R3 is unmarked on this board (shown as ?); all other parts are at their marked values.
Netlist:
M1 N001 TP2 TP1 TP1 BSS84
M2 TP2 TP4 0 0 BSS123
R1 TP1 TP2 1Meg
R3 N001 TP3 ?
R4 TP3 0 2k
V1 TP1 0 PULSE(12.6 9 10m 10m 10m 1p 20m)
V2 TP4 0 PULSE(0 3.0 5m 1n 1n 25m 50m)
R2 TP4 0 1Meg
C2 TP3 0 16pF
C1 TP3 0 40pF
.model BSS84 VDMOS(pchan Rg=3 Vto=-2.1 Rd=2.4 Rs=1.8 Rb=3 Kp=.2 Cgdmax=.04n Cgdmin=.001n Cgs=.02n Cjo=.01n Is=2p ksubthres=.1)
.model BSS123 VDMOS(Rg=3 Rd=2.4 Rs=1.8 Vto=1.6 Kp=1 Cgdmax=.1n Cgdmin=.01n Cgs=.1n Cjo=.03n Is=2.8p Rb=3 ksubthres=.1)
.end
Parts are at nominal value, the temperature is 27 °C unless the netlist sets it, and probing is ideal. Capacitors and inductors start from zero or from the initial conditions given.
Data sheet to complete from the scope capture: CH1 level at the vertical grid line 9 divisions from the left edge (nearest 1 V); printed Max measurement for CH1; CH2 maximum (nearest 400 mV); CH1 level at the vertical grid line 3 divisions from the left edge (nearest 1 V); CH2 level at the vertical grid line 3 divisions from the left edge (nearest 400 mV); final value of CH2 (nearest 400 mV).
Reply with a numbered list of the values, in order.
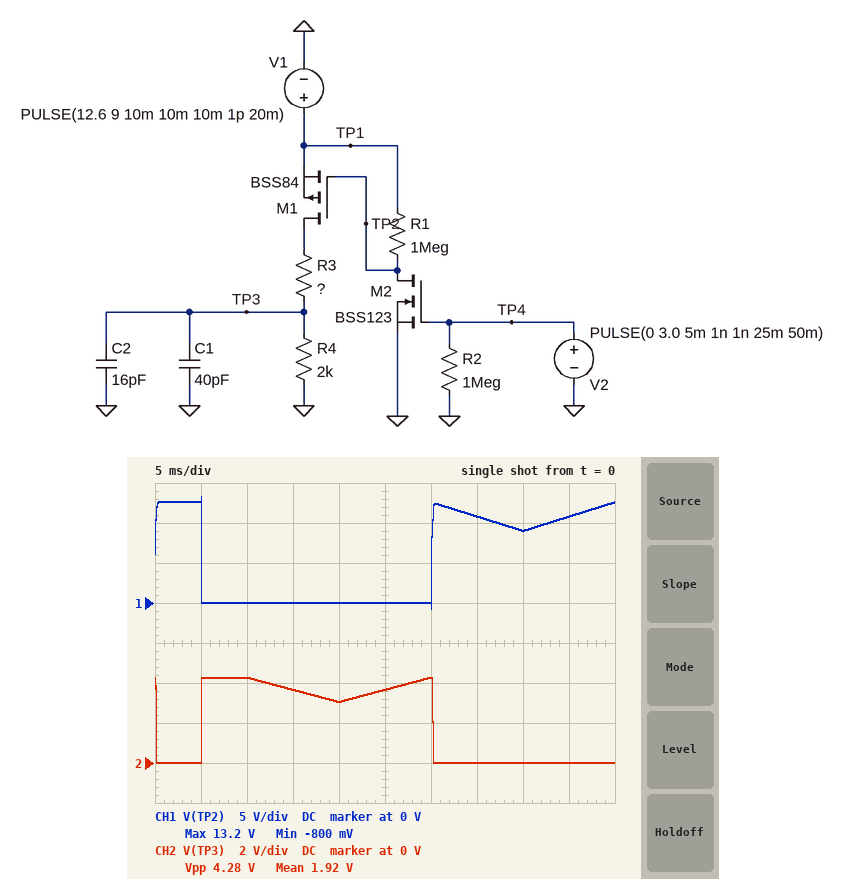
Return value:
1. 11 V
2. 13.2 V
3. 4.4 V
4. 0 V
5. 3.6 V
6. 0 V
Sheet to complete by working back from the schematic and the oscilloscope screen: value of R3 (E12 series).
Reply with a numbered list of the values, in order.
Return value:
1. 3.9 kΩ
